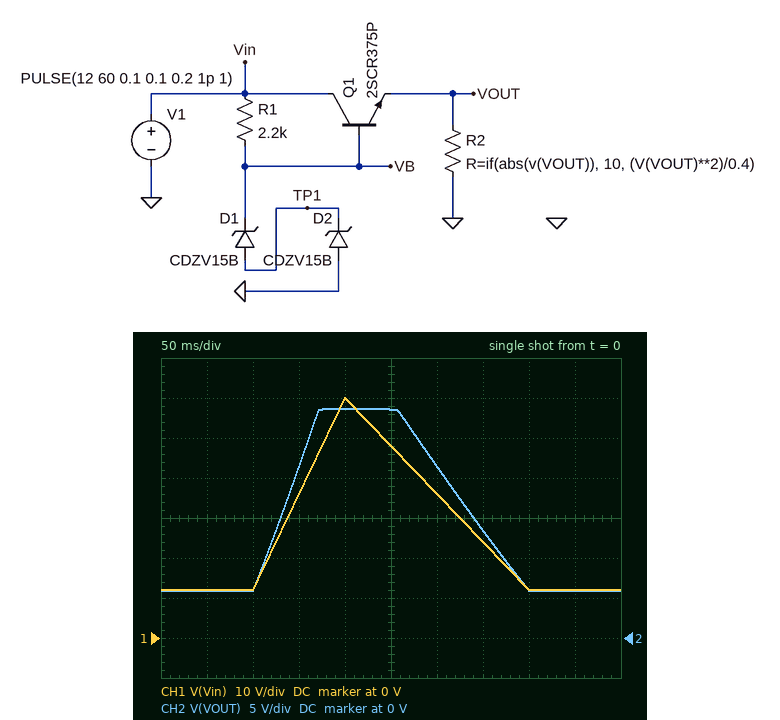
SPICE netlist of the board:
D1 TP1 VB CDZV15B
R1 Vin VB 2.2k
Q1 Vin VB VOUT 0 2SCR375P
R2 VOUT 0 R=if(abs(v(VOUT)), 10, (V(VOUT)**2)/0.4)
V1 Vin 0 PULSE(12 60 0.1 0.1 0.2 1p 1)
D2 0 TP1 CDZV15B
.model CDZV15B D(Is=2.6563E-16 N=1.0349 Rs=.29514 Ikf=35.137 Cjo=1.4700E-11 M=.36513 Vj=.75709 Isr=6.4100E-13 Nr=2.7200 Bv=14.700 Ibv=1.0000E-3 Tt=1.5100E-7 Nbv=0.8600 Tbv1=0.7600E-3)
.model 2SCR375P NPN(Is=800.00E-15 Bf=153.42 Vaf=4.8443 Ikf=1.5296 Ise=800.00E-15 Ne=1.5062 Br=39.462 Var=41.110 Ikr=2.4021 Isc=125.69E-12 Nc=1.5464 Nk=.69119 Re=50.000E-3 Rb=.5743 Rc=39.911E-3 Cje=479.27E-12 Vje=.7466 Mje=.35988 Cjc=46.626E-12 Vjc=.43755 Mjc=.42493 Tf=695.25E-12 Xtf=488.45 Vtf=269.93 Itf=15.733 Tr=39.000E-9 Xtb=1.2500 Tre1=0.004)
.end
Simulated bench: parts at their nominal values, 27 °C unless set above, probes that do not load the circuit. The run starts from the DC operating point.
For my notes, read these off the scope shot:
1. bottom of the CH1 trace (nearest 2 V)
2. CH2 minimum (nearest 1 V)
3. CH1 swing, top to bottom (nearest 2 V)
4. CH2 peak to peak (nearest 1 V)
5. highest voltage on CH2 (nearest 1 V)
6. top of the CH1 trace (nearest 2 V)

12 V
6 V
48 V
23 V
29 V
60 V
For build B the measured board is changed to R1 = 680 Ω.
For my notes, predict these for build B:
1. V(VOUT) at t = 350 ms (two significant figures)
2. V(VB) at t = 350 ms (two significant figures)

17 V
18 V
